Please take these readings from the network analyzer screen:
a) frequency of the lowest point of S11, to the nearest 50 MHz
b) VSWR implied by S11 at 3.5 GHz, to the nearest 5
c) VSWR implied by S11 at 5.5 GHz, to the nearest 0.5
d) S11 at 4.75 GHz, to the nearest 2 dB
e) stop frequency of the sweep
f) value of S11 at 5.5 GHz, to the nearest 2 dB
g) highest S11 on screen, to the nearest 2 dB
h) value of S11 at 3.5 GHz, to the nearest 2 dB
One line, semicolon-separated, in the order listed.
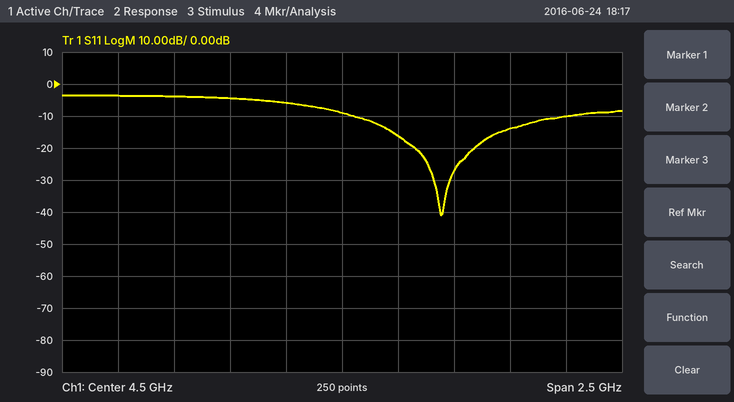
4.95 GHz; 5; 2.0; -16 dB; 5.75 GHz; -10 dB; -4 dB; -4 dB
